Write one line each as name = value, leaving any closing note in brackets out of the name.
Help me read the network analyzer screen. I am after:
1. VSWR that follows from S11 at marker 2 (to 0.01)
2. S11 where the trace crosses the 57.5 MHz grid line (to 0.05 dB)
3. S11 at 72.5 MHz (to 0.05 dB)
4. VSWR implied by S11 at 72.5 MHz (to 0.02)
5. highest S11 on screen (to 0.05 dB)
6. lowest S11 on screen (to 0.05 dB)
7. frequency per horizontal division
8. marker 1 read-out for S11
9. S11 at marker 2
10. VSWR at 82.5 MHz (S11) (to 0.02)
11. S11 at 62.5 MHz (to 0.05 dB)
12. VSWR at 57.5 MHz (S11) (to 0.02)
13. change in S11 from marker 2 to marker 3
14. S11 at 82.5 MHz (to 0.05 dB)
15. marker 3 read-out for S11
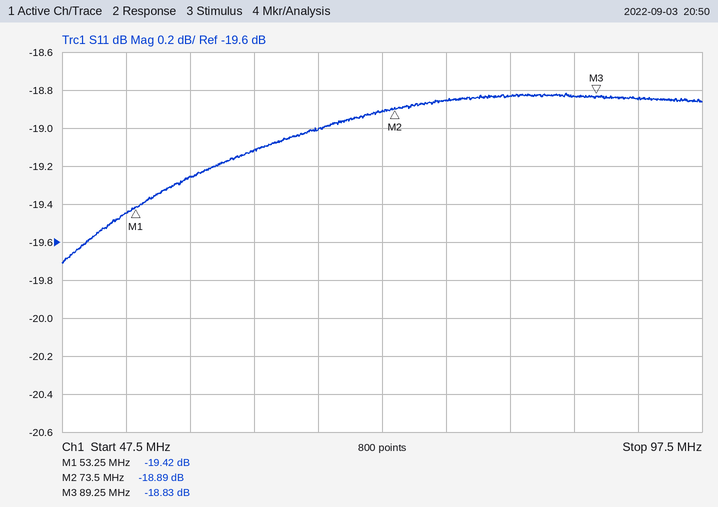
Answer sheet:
VSWR that follows from S11 at marker 2 = 1.26
S11 where the trace crosses the 57.5 MHz grid line = -19.25 dB
S11 at 72.5 MHz = -18.90 dB
VSWR implied by S11 at 72.5 MHz = 1.26
highest S11 on screen = -18.80 dB
lowest S11 on screen = -19.70 dB
frequency per horizontal division = 5 MHz
marker 1 read-out for S11 = -19.42 dB
S11 at marker 2 = -18.89 dB
VSWR at 82.5 MHz (S11) = 1.26
S11 at 62.5 MHz = -19.10 dB
VSWR at 57.5 MHz (S11) = 1.24
change in S11 from marker 2 to marker 3 = 0.06 dB
S11 at 82.5 MHz = -18.85 dB
marker 3 read-out for S11 = -18.83 dB
